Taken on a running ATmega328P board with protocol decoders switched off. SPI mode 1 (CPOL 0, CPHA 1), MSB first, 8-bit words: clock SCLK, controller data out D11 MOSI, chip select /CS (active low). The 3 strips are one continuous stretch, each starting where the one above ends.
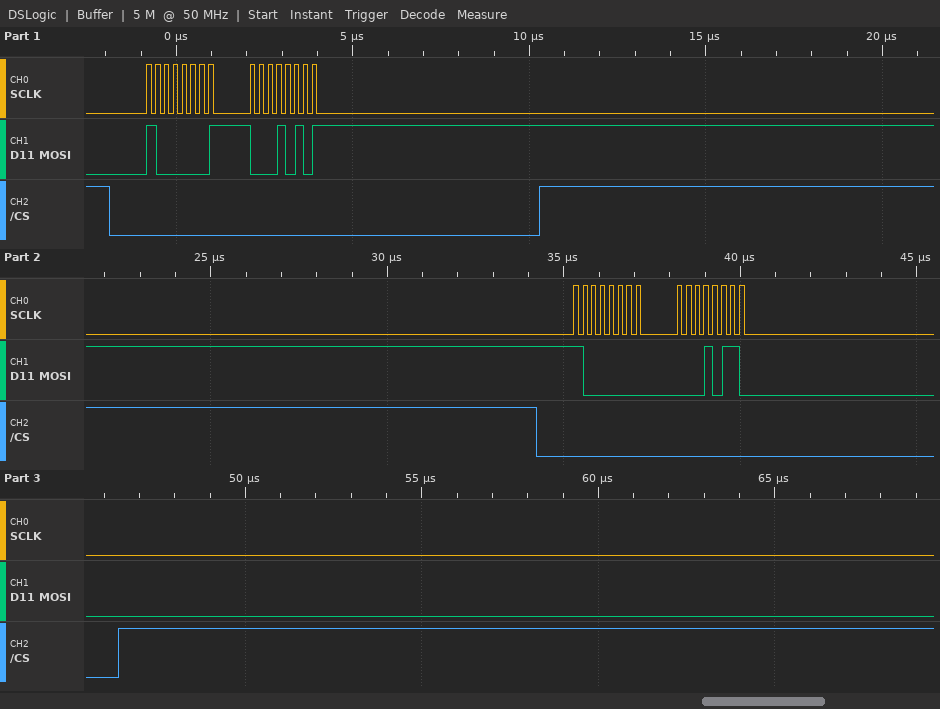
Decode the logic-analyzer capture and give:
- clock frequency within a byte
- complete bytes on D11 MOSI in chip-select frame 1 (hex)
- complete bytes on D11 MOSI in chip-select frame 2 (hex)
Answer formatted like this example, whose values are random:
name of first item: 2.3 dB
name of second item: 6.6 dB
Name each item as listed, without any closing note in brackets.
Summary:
clock frequency within a byte: 4 MHz
complete bytes on D11 MOSI in chip-select frame 1: 81 15
complete bytes on D11 MOSI in chip-select frame 2: 80 16
